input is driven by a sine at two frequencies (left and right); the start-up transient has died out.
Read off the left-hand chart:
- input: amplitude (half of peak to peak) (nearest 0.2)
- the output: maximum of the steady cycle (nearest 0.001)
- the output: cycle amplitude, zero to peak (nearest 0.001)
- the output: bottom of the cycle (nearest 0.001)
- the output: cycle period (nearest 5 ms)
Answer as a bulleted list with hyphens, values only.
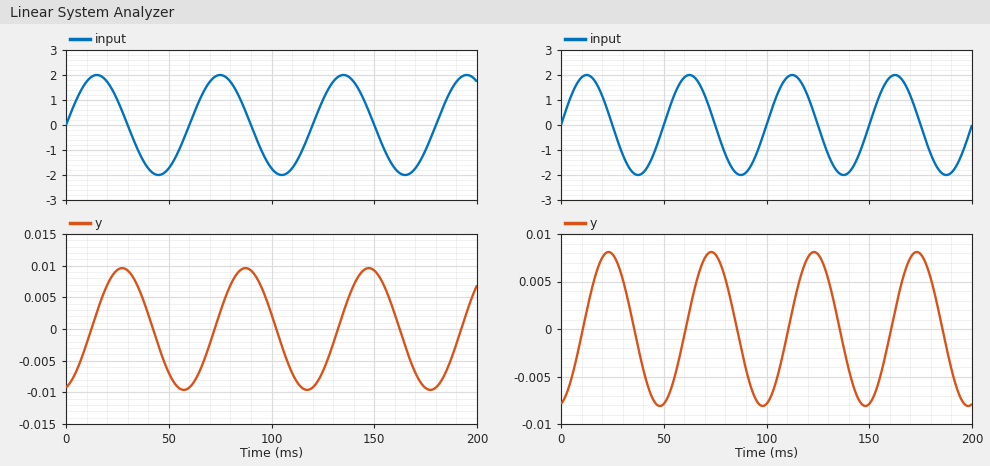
- 2.0
- 0.010
- 0.010
- -0.010
- 60 ms
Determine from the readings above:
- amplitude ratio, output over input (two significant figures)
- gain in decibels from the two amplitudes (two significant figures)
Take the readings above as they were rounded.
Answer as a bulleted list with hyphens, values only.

- 0.0050
- -46 dB
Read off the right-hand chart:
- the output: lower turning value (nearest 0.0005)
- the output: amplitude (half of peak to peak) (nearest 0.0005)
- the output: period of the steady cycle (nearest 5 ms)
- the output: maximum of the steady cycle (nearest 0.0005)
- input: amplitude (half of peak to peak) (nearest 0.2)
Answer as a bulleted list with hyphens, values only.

- -0.0080
- 0.0080
- 50 ms
- 0.0080
- 2.0
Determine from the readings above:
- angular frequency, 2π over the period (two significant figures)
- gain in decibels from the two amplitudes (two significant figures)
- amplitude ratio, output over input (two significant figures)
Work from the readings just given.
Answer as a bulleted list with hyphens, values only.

- 0.13 rad/ms
- -48 dB
- 0.0040
